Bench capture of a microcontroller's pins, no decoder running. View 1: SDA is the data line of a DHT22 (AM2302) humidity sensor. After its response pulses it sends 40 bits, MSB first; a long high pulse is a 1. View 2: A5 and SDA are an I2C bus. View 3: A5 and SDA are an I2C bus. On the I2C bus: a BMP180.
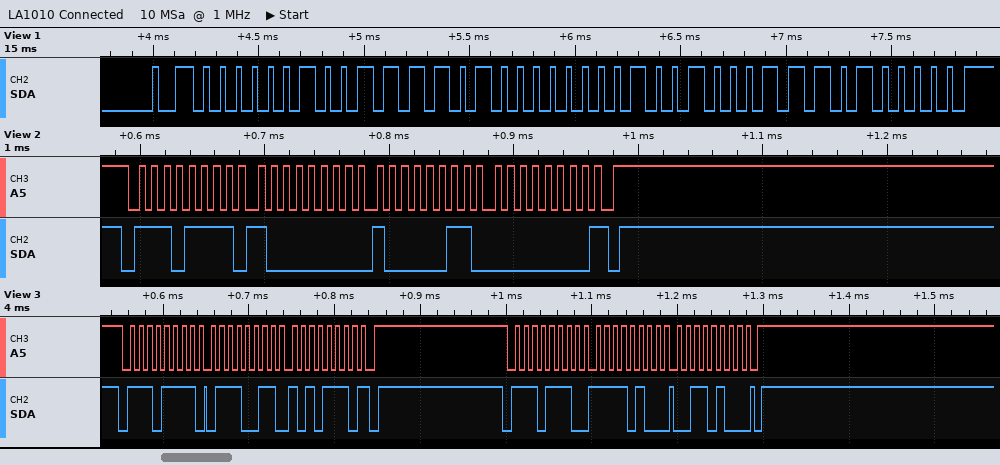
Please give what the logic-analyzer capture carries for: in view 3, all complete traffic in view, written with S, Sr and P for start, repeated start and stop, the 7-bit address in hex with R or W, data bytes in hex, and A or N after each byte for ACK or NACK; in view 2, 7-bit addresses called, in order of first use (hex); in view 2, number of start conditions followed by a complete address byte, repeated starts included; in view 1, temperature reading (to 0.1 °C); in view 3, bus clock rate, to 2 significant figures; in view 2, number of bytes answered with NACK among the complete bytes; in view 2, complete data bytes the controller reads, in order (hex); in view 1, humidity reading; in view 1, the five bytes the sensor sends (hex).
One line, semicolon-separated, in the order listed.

S 77R A 73 A AE N P S 77W A F4 A 34 A P; 0x77; 1; 29.1 °C; 100 kHz; 1; 80 83 00; 63.4 %; 02 7A 01 23 A0
